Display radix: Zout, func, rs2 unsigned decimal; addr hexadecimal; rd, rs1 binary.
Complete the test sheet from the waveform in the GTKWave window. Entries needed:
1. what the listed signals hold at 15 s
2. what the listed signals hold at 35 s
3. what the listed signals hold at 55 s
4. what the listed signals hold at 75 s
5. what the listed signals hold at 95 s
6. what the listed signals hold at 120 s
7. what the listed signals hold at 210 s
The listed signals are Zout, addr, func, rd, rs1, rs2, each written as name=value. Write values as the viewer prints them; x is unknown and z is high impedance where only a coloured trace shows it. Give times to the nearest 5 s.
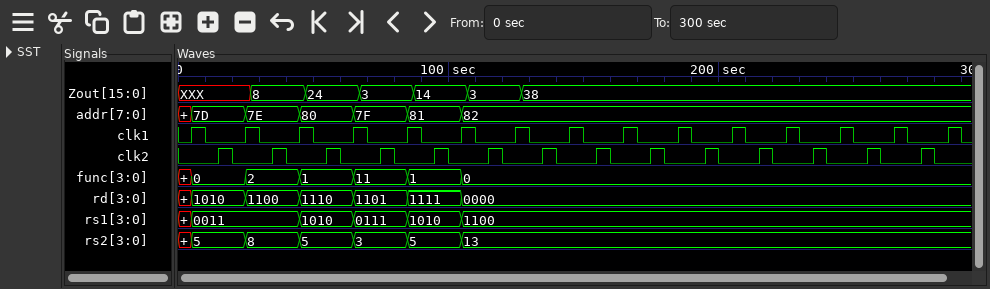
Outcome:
Zout=XXX, addr=7D, func=0, rd=1010, rs1=0011, rs2=5
Zout=8, addr=7E, func=2, rd=1100, rs1=0011, rs2=8
Zout=24, addr=80, func=1, rd=1110, rs1=1010, rs2=5
Zout=3, addr=7F, func=11, rd=1101, rs1=0111, rs2=3
Zout=14, addr=81, func=1, rd=1111, rs1=1010, rs2=5
Zout=3, addr=82, func=0, rd=0000, rs1=1100, rs2=13
Zout=38, addr=82, func=0, rd=0000, rs1=1100, rs2=13
